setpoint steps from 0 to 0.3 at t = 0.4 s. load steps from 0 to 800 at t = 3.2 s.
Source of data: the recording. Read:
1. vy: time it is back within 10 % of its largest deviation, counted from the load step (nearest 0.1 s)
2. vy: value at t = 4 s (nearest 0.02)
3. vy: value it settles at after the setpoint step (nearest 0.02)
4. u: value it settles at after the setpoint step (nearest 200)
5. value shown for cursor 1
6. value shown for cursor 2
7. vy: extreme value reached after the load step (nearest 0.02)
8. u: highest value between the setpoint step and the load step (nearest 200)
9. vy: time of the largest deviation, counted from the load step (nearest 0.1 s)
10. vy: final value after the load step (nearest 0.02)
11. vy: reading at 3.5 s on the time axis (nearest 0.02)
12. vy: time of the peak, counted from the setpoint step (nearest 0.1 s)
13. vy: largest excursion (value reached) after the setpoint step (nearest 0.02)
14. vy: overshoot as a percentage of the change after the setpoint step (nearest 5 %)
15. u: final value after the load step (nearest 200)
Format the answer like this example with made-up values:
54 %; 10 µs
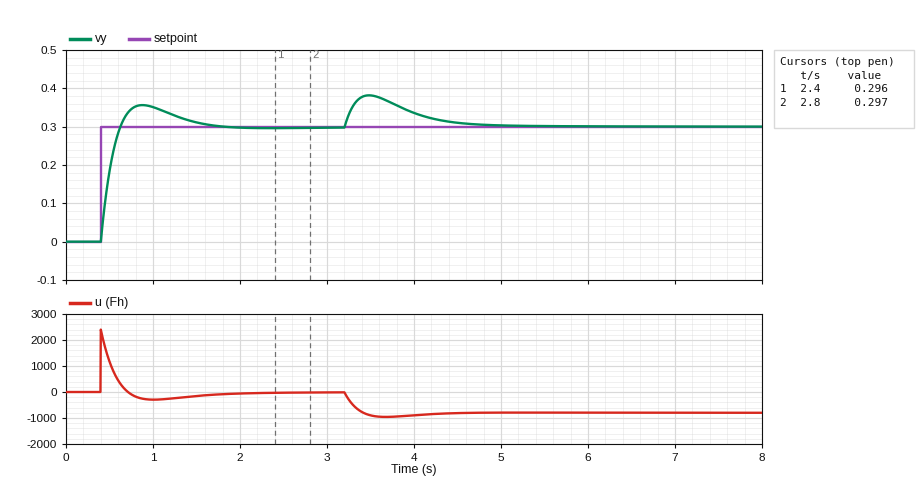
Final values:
1.4 s; 0.34; 0.30; 0; 0.296; 0.297; 0.38; 2400; 0.3 s; 0.30; 0.38; 0.5 s; 0.36; 20 %; -800
